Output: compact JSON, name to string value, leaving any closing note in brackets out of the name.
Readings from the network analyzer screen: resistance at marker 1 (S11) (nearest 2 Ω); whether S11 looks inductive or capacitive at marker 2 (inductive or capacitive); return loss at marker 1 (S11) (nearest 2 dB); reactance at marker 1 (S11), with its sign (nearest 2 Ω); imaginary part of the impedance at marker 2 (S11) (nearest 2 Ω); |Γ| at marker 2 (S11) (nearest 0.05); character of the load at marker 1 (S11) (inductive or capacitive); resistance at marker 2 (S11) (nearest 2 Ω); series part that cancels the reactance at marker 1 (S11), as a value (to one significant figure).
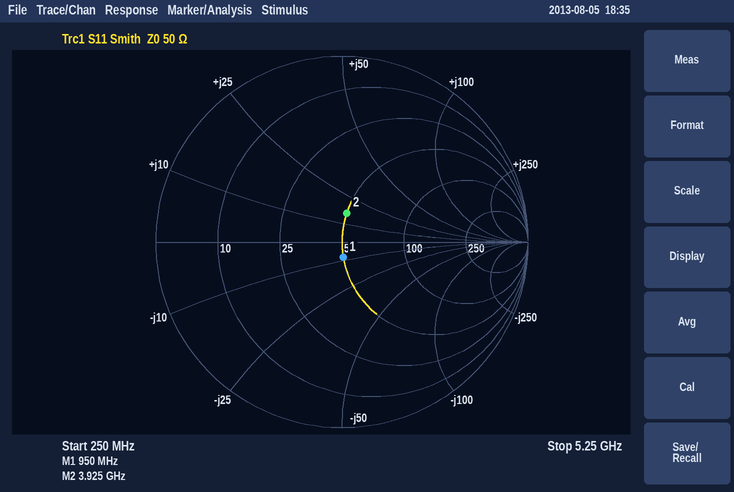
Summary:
{"resistance at marker 1 (S11)": "50 Ω", "whether S11 looks inductive or capacitive at marker 2": "inductive", "return loss at marker 1 (S11)": "22 dB", "reactance at marker 1 (S11), with its sign": "-8 Ω", "imaginary part of the impedance at marker 2 (S11)": "+16 Ω", "|Γ| at marker 2 (S11)": "0.15", "character of the load at marker 1 (S11)": "capacitive", "resistance at marker 2 (S11)": "50 Ω", "series part that cancels the reactance at marker 1 (S11), as a value": "1 nH"}
